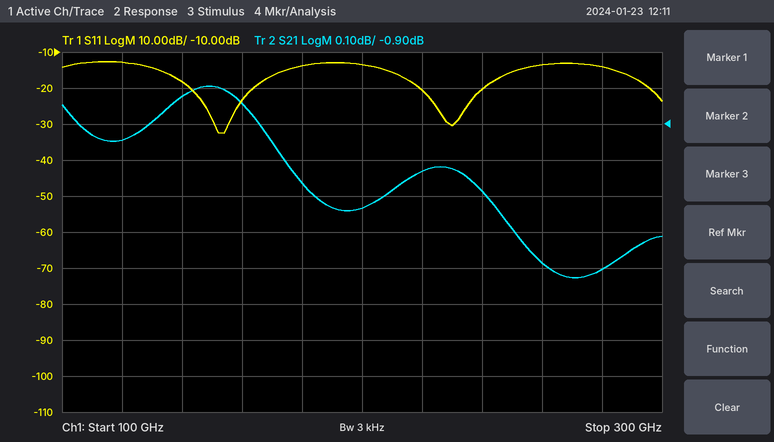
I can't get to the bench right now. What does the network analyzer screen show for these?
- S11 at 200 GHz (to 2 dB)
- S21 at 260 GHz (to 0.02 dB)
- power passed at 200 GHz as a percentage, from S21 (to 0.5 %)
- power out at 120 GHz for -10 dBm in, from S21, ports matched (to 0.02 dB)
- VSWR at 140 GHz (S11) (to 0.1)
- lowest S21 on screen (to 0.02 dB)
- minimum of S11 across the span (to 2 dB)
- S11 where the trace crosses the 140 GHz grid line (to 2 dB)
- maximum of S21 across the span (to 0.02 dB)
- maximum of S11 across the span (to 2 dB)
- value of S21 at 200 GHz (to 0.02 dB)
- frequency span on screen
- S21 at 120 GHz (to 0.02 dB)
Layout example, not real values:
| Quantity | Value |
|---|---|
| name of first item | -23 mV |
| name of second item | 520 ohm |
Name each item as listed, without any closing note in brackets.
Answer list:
| Quantity | Value |
|---|---|
| S11 at 200 GHz | -14 dB |
| S21 at 260 GHz | -1.28 dB |
| power passed at 200 GHz as a percentage, from S21 | 77.0 % |
| power out at 120 GHz for -10 dBm in, from S21, ports matched | -10.94 dBm |
| VSWR at 140 GHz (S11) | 1.3 |
| lowest S21 on screen | -1.32 dB |
| minimum of S11 across the span | -32 dB |
| S11 where the trace crosses the 140 GHz grid line | -18 dB |
| maximum of S21 across the span | -0.80 dB |
| maximum of S11 across the span | -12 dB |
| value of S21 at 200 GHz | -1.14 dB |
| frequency span on screen | 200 GHz |
| S21 at 120 GHz | -0.94 dB |
